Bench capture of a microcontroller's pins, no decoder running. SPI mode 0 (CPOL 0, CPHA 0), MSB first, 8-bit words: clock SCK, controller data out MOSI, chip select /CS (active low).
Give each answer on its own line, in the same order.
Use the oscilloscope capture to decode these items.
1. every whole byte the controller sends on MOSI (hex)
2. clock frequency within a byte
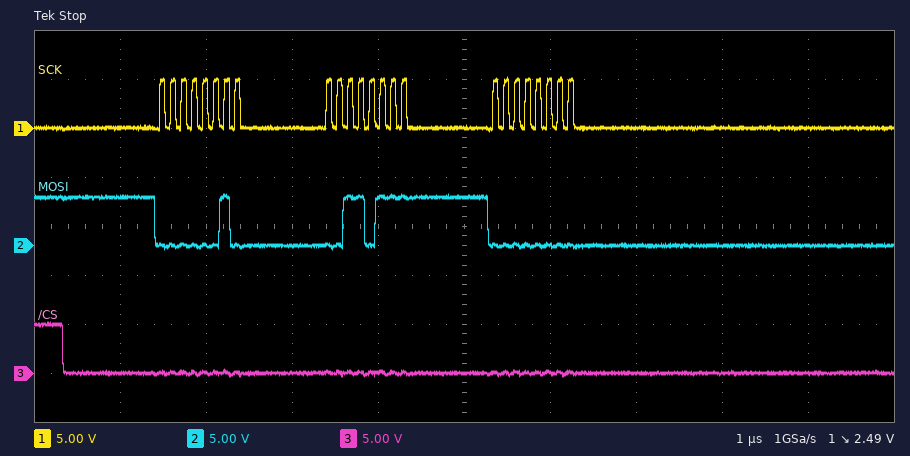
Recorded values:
02 37 00
8 MHz
